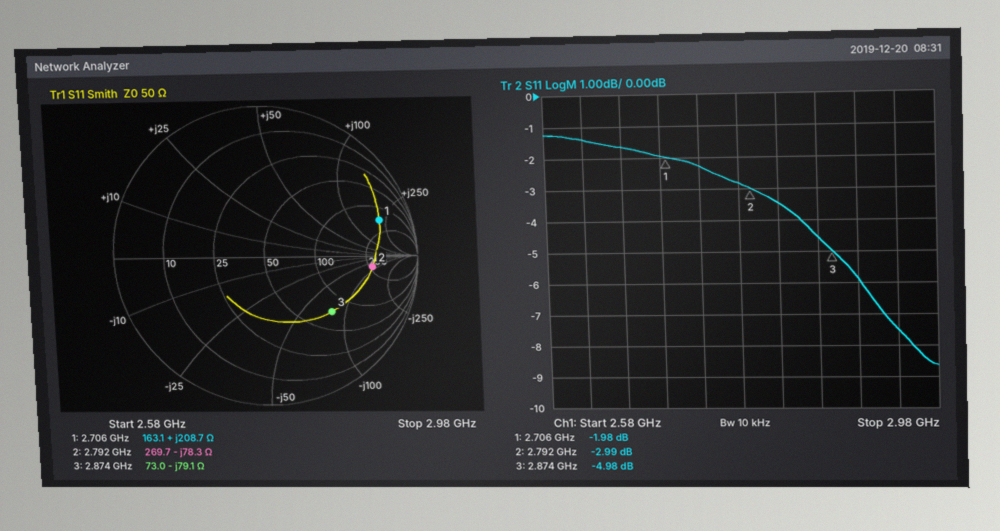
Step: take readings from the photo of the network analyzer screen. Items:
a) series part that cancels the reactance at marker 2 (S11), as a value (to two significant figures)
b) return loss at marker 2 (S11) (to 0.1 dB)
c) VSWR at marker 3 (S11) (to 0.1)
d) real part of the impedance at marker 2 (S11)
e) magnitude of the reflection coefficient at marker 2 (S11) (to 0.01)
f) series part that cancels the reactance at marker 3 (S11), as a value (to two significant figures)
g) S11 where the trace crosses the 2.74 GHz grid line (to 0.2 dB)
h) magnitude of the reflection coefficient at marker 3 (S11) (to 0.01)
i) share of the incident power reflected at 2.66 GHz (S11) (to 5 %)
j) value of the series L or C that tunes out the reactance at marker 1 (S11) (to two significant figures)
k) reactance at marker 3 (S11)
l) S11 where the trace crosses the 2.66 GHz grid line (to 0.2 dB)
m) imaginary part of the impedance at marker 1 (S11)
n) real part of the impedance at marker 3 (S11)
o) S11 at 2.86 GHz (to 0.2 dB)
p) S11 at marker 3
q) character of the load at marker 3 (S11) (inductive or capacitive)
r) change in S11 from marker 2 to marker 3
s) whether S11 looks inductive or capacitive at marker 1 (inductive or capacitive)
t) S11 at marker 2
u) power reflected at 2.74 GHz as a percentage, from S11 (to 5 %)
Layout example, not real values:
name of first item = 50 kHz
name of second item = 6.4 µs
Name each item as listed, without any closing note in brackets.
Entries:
series part that cancels the reactance at marker 2 (S11), as a value = 4.5 nH
return loss at marker 2 (S11) = 3.0 dB
VSWR at marker 3 (S11) = 3.6
real part of the impedance at marker 2 = 269.7 Ω
magnitude of the reflection coefficient at marker 2 (S11) = 0.71
series part that cancels the reactance at marker 3 (S11), as a value = 4.4 nH
S11 where the trace crosses the 2.74 GHz grid line = -2.2 dB
magnitude of the reflection coefficient at marker 3 (S11) = 0.56
share of the incident power reflected at 2.66 GHz (S11) = 70 %
value of the series L or C that tunes out the reactance at marker 1 (S11) = 280 fF
reactance at marker 3 = -79.1 Ω
S11 where the trace crosses the 2.66 GHz grid line = -1.6 dB
imaginary part of the impedance at marker 1 = +208.7 Ω
real part of the impedance at marker 3 = 73.0 Ω
S11 at 2.86 GHz = -4.6 dB
S11 at marker 3 = -4.98 dB
character of the load at marker 3 (S11) = capacitive
change in S11 from marker 2 to marker 3 = -1.99 dB
whether S11 looks inductive or capacitive at marker 1 = inductive
S11 at marker 2 = -2.99 dB
power reflected at 2.74 GHz as a percentage, from S11 = 60 %
